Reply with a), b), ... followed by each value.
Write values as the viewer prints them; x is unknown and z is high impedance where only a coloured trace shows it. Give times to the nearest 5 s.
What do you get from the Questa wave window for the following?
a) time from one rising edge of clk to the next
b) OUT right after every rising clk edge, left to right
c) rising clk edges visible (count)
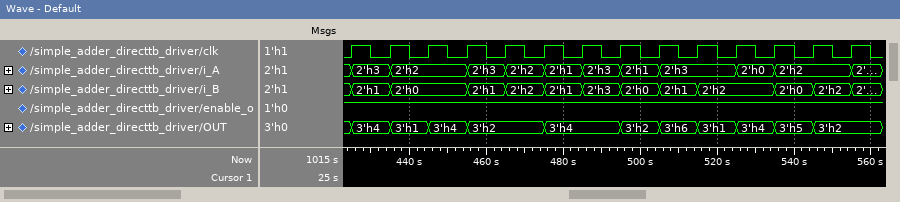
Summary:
a) 10 s
b) 3'h4, 3'h1, 3'h4, 3'h2, 3'h2, 3'h4, 3'h4, 3'h2, 3'h6, 3'h1, 3'h4, 3'h5, 3'h2, 3'h2
c) 14
